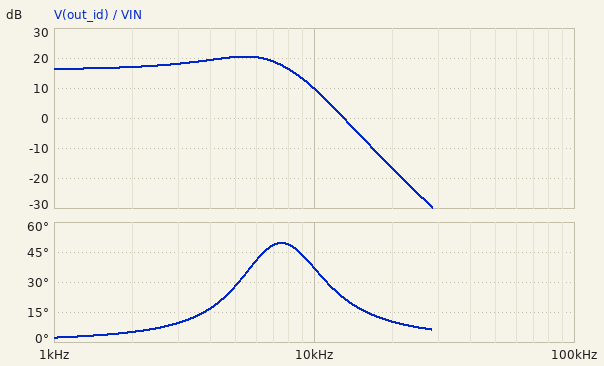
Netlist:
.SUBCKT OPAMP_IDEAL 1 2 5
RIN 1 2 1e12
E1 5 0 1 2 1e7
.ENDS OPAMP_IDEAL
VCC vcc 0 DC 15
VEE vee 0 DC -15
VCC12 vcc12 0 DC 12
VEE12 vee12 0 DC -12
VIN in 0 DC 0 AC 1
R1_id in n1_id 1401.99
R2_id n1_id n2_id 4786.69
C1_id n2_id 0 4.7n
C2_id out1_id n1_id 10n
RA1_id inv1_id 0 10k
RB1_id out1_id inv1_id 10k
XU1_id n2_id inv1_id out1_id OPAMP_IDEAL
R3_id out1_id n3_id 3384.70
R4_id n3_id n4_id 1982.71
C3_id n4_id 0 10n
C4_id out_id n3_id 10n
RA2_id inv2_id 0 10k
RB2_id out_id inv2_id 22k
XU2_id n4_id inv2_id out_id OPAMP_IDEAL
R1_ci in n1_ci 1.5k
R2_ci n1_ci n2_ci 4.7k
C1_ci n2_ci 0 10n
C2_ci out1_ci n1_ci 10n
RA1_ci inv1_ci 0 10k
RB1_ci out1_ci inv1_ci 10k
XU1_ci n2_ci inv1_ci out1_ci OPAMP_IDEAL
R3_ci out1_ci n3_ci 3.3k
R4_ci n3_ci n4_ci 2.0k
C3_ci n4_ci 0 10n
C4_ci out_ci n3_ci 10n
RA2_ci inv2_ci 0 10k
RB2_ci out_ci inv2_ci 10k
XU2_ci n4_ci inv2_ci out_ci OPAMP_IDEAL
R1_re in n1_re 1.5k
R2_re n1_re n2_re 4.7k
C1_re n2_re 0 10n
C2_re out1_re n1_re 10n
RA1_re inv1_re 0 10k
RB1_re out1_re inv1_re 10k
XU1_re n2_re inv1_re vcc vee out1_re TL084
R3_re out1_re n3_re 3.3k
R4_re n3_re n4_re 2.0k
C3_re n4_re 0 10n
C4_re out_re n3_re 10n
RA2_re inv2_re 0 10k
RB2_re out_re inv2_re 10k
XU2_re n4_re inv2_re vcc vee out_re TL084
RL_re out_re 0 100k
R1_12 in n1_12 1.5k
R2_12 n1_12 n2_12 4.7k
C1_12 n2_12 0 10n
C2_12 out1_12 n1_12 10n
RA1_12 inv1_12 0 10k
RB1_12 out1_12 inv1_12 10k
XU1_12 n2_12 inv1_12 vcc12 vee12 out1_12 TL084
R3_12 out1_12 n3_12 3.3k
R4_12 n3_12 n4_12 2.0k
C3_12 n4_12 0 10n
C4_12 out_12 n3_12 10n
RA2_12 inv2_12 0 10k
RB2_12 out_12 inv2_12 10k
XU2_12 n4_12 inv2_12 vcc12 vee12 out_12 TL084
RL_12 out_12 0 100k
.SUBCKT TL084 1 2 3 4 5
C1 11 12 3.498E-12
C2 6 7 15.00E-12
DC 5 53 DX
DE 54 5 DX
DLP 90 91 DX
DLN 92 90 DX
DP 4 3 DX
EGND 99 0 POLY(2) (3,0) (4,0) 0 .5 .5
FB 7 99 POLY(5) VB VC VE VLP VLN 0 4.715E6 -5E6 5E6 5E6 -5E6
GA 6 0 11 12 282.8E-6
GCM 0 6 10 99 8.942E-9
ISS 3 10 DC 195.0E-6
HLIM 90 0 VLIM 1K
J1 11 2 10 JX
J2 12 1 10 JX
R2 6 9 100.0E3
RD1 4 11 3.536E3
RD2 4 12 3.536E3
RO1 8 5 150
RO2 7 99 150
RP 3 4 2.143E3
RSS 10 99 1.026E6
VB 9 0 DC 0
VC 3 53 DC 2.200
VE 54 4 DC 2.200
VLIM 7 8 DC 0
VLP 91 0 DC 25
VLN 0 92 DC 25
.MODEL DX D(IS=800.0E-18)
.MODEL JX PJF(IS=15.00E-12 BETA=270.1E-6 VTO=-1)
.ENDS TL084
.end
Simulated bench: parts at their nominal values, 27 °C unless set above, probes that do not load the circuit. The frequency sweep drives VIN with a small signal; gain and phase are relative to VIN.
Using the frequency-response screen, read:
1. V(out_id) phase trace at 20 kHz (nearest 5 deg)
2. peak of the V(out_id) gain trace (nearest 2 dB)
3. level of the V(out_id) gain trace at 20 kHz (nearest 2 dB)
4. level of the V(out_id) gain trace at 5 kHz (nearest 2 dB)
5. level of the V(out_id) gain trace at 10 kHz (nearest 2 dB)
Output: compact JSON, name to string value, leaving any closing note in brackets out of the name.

{"V(out_id) phase trace at 20 kHz": "10 deg", "peak of the V(out_id) gain trace": "20 dB", "level of the V(out_id) gain trace at 20 kHz": "-16 dB", "level of the V(out_id) gain trace at 5 kHz": "20 dB", "level of the V(out_id) gain trace at 10 kHz": "10 dB"}
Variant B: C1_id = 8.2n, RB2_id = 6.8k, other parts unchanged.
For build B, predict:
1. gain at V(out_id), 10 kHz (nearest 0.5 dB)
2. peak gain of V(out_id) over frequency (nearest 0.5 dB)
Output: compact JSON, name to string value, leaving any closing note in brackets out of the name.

{"gain at V(out_id), 10 kHz": "-6.0 dB", "peak gain of V(out_id) over frequency": "10.5 dB"}
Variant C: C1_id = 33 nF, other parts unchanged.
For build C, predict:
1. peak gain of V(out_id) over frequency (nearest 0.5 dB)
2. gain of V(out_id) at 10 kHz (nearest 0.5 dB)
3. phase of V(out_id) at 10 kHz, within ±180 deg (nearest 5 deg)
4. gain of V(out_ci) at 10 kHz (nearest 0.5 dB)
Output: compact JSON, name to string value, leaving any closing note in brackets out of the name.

{"peak gain of V(out_id) over frequency": "16.0 dB", "gain of V(out_id) at 10 kHz": "-13.5 dB", "phase of V(out_id) at 10 kHz, within ±180 deg": "20 deg", "gain of V(out_ci) at 10 kHz": "-5.0 dB"}
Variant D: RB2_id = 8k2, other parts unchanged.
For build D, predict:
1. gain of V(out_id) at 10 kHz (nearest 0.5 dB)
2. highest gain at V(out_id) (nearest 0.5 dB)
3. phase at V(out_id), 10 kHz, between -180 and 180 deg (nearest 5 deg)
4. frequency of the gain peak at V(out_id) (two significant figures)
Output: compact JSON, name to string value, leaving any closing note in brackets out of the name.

{"gain of V(out_id) at 10 kHz": "4.0 dB", "highest gain at V(out_id)": "14.0 dB", "phase at V(out_id), 10 kHz, between -180 and 180 deg": "120 deg", "frequency of the gain peak at V(out_id)": "5.0 kHz"}
